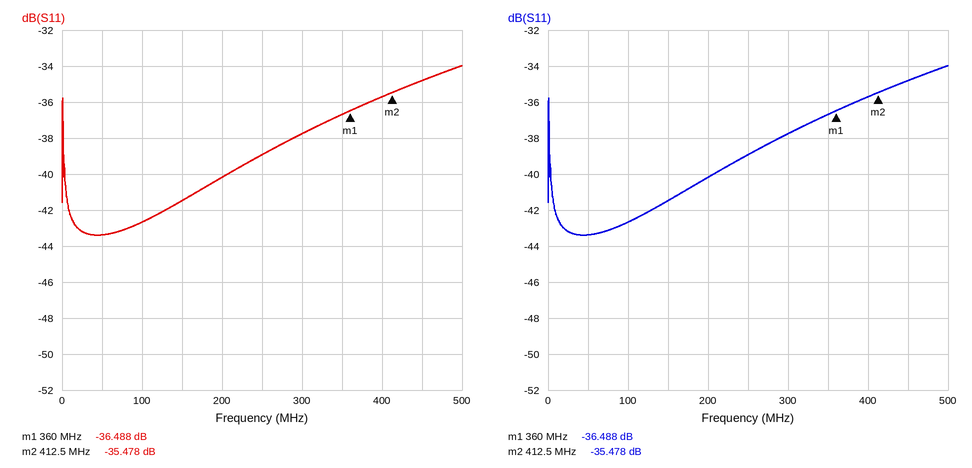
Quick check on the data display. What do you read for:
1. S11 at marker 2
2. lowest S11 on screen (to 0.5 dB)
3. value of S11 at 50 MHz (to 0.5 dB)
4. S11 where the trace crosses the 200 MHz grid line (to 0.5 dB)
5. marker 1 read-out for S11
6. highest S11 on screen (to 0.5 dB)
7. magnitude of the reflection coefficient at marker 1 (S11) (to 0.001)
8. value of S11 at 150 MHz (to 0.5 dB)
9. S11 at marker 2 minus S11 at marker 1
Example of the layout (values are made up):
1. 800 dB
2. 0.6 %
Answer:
1. -35.478 dB
2. -43.5 dB
3. -43.5 dB
4. -40.0 dB
5. -36.488 dB
6. -34.0 dB
7. 0.015
8. -41.5 dB
9. 1.010 dB
